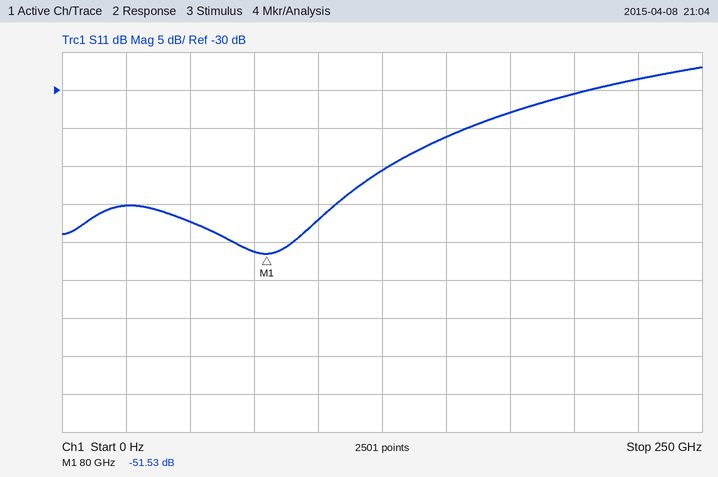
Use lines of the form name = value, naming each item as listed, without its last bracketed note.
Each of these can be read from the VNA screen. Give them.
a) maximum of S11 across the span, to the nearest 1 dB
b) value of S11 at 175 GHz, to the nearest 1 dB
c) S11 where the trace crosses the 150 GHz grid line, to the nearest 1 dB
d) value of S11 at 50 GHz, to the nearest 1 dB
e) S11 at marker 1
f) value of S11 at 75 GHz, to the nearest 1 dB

maximum of S11 across the span, to the nearest 1 dB = -27 dB
value of S11 at 175 GHz, to the nearest 1 dB = -33 dB
S11 where the trace crosses the 150 GHz grid line, to the nearest 1 dB = -36 dB
value of S11 at 50 GHz, to the nearest 1 dB = -47 dB
S11 at marker 1 = -51.53 dB
value of S11 at 75 GHz, to the nearest 1 dB = -51 dB
